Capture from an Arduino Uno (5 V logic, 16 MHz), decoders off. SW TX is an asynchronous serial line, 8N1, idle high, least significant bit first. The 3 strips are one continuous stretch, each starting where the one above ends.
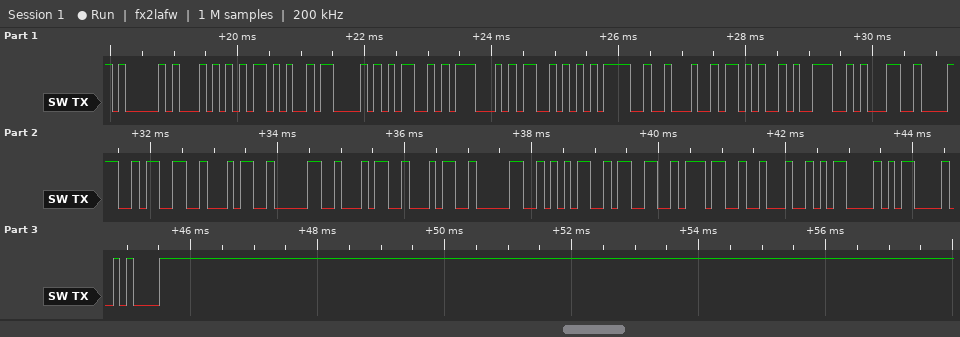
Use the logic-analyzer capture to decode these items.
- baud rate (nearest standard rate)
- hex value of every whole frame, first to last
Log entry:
9600 baud
41 54 2B 43 4D 47 53 3D 22 2B 39 31 38 33 34 30 34 34 30 35 33 37 22 0D 0D 0A
